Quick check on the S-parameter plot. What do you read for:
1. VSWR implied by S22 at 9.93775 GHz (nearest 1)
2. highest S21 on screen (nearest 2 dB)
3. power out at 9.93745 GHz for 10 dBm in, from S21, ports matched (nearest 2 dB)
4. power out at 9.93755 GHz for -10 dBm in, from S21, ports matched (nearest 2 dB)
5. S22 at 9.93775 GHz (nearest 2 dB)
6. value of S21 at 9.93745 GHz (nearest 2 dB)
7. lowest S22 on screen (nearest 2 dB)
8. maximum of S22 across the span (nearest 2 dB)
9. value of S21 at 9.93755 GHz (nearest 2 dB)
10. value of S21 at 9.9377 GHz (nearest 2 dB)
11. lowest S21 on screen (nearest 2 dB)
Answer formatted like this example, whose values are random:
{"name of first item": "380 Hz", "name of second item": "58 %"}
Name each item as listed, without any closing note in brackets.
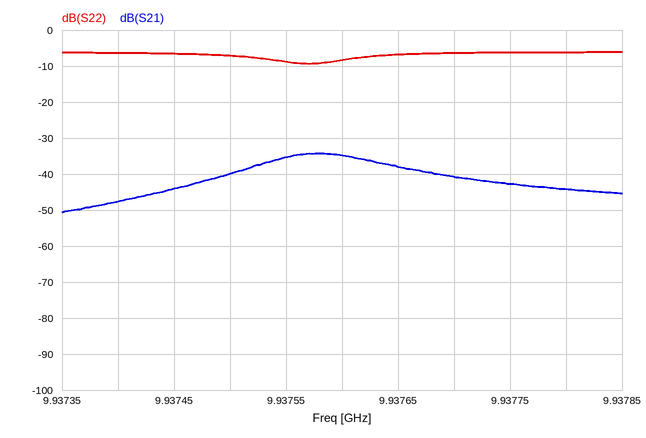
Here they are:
{"VSWR implied by S22 at 9.93775 GHz": "3", "highest S21 on screen": "-34 dB", "power out at 9.93745 GHz for 10 dBm in, from S21, ports matched": "-34 dBm", "power out at 9.93755 GHz for -10 dBm in, from S21, ports matched": "-46 dBm", "S22 at 9.93775 GHz": "-6 dB", "value of S21 at 9.93745 GHz": "-44 dB", "lowest S22 on screen": "-10 dB", "maximum of S22 across the span": "-6 dB", "value of S21 at 9.93755 GHz": "-36 dB", "value of S21 at 9.9377 GHz": "-40 dB", "lowest S21 on screen": "-50 dB"}
